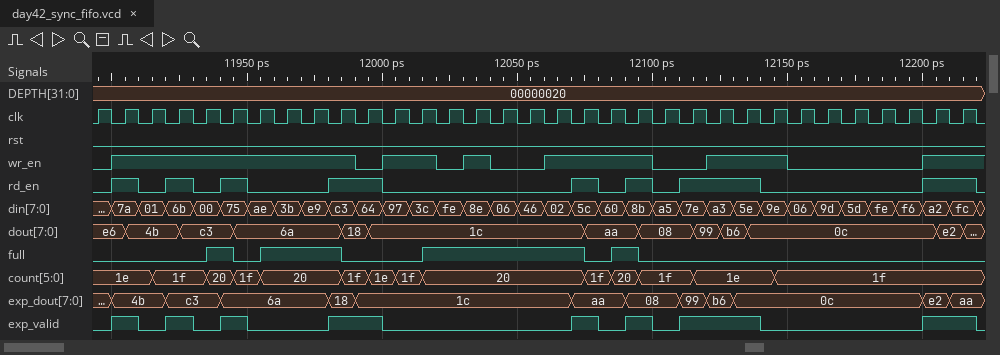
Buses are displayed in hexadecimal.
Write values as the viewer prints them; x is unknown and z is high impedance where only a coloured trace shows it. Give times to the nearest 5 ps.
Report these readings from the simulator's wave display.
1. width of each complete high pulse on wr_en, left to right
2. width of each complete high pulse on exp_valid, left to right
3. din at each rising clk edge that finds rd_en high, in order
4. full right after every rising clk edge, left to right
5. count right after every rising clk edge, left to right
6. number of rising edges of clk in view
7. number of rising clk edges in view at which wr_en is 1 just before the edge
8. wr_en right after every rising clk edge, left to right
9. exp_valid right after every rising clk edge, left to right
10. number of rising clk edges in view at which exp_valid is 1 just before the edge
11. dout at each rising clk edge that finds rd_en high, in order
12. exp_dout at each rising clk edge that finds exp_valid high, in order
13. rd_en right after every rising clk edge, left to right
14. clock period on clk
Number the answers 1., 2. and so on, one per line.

1. 90 ps, 20 ps, 10 ps, 40 ps, 30 ps
2. 10 ps, 10 ps, 10 ps, 20 ps, 10 ps, 10 ps, 30 ps, 20 ps
3. 7a, 6b, 75, c3, 64, 5c, 8b, 7e, a3, 5e, a2, fc
4. 0 0 0 0 1 0 1 1 1 0 0 0 1 1 1 1 1 1 0 1 0 0 0 0 0 0 0 0 0 0 0 0 0
5. 1e, 1e, 1f, 1f, 20, 1f, 20, 20, 20, 1f, 1e, 1f, 20, 20, 20, 20, 20, 20, 1f, 20, 1f, 1f, 1e, 1e, 1e, 1f, 1f, 1f, 1f, 1f, 1f, 1f, 1f
6. 33
7. 21
8. 0 1 1 1 1 1 1 1 1 1 0 1 1 0 1 0 0 1 1 1 1 0 0 1 1 1 0 0 0 0 0 1 1
9. 0 1 0 1 0 1 0 0 0 1 1 0 0 0 0 0 0 0 1 0 1 0 1 1 1 0 0 0 0 0 0 1 1
10. 12
11. e6, 4b, c3, 6a, 18, 1c, aa, 08, 99, b6, 0c, e2
12. 4b, c3, 6a, 18, 1c, aa, 08, 99, b6, 0c, e2, aa
13. 0 1 0 1 0 1 0 0 0 1 1 0 0 0 0 0 0 0 1 0 1 0 1 1 1 0 0 0 0 0 0 1 1
14. 10 ps
